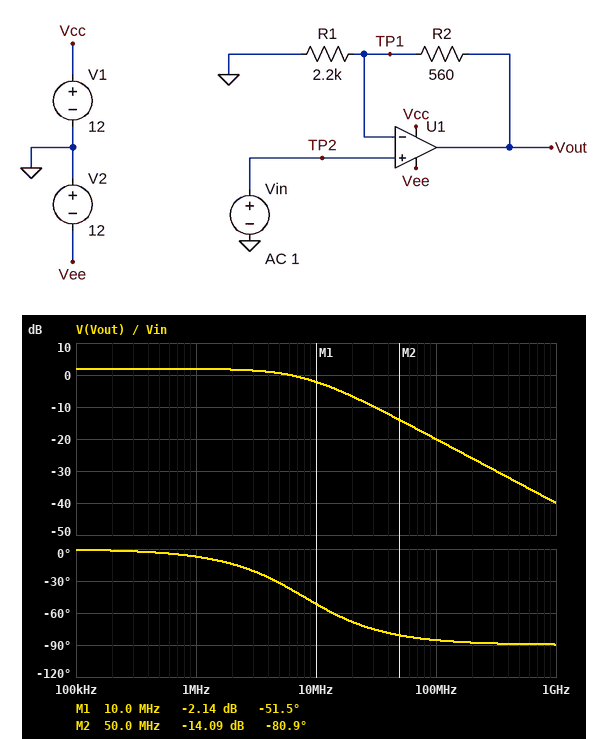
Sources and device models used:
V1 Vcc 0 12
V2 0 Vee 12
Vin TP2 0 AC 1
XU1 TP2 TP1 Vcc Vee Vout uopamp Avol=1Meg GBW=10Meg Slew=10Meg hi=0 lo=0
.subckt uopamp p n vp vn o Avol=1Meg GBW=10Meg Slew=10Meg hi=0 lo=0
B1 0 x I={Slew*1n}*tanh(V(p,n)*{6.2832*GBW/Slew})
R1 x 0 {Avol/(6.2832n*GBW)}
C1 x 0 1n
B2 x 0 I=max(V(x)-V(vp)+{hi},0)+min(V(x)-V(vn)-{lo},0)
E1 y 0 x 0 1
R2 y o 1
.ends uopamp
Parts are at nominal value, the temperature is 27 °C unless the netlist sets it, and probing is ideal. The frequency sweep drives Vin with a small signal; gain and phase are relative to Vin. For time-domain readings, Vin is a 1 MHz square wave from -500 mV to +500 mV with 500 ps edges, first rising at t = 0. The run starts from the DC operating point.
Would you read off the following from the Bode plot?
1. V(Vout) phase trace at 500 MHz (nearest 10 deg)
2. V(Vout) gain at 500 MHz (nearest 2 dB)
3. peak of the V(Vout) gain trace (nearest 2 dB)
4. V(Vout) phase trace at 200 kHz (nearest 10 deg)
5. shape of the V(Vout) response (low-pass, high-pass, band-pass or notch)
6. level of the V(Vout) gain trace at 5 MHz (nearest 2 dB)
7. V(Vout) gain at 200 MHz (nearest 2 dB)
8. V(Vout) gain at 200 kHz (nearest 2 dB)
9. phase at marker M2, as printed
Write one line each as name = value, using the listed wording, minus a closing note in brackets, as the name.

V(Vout) phase trace at 500 MHz = -90 deg
V(Vout) gain at 500 MHz = -34 dB
peak of the V(Vout) gain trace = 2 dB
V(Vout) phase trace at 200 kHz = 0 deg
shape of the V(Vout) response = low-pass
level of the V(Vout) gain trace at 5 MHz = 0 dB
V(Vout) gain at 200 MHz = -26 dB
V(Vout) gain at 200 kHz = 2 dB
phase at marker M2, as printed = -80.9 deg
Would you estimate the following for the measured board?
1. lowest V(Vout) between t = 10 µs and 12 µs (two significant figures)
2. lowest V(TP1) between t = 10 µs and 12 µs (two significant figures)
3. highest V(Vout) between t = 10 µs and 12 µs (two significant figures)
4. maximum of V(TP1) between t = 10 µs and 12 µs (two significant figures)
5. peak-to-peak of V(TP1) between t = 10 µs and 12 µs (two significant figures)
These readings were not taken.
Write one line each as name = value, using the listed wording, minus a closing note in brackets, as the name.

lowest V(Vout) between t = 10 µs and 12 µs = -630 mV
lowest V(TP1) between t = 10 µs and 12 µs = -500 mV
highest V(Vout) between t = 10 µs and 12 µs = 630 mV
maximum of V(TP1) between t = 10 µs and 12 µs = 500 mV
peak-to-peak of V(TP1) between t = 10 µs and 12 µs = 1.0 V
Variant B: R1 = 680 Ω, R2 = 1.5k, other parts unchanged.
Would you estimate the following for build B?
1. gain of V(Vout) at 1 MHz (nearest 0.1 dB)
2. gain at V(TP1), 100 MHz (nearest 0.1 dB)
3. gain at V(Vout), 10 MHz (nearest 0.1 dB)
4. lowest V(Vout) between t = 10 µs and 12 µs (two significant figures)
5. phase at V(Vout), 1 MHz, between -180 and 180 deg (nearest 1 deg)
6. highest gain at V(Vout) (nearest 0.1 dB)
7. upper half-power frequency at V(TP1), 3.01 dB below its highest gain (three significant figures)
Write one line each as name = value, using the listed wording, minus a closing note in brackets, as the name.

gain of V(Vout) at 1 MHz = 9.7 dB
gain at V(TP1), 100 MHz = -30.1 dB
gain at V(Vout), 10 MHz = -0.4 dB
lowest V(Vout) between t = 10 µs and 12 µs = -1.6 V
phase at V(Vout), 1 MHz, between -180 and 180 deg = -18 deg
highest gain at V(Vout) = 10.1 dB
upper half-power frequency at V(TP1), 3.01 dB below its highest gain = 3.12 MHz
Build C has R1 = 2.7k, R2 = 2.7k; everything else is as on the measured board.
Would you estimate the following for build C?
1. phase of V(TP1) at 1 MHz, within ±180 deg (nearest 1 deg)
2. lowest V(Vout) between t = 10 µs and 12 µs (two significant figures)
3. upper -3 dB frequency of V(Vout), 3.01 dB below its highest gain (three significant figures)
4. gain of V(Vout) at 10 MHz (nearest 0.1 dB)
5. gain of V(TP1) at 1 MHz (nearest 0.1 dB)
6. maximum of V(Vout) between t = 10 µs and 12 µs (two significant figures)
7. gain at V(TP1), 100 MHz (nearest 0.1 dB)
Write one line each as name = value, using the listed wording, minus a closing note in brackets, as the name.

phase of V(TP1) at 1 MHz, within ±180 deg = -11 deg
lowest V(Vout) between t = 10 µs and 12 µs = -1.0 V
upper -3 dB frequency of V(Vout), 3.01 dB below its highest gain = 5.00 MHz
gain of V(Vout) at 10 MHz = -1.0 dB
gain of V(TP1) at 1 MHz = -0.2 dB
maximum of V(Vout) between t = 10 µs and 12 µs = 1.0 V
gain at V(TP1), 100 MHz = -26.0 dB
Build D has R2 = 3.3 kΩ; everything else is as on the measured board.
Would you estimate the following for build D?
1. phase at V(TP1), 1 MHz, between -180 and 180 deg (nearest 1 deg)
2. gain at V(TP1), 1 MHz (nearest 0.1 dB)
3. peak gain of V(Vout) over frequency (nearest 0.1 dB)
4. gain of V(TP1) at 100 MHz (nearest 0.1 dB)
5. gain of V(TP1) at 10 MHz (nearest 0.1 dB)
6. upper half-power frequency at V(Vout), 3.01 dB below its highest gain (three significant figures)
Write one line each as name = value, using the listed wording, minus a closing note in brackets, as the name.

phase at V(TP1), 1 MHz, between -180 and 180 deg = -14 deg
gain at V(TP1), 1 MHz = -0.3 dB
peak gain of V(Vout) over frequency = 8.0 dB
gain of V(TP1) at 100 MHz = -28.0 dB
gain of V(TP1) at 10 MHz = -8.6 dB
upper half-power frequency at V(Vout), 3.01 dB below its highest gain = 4.00 MHz
